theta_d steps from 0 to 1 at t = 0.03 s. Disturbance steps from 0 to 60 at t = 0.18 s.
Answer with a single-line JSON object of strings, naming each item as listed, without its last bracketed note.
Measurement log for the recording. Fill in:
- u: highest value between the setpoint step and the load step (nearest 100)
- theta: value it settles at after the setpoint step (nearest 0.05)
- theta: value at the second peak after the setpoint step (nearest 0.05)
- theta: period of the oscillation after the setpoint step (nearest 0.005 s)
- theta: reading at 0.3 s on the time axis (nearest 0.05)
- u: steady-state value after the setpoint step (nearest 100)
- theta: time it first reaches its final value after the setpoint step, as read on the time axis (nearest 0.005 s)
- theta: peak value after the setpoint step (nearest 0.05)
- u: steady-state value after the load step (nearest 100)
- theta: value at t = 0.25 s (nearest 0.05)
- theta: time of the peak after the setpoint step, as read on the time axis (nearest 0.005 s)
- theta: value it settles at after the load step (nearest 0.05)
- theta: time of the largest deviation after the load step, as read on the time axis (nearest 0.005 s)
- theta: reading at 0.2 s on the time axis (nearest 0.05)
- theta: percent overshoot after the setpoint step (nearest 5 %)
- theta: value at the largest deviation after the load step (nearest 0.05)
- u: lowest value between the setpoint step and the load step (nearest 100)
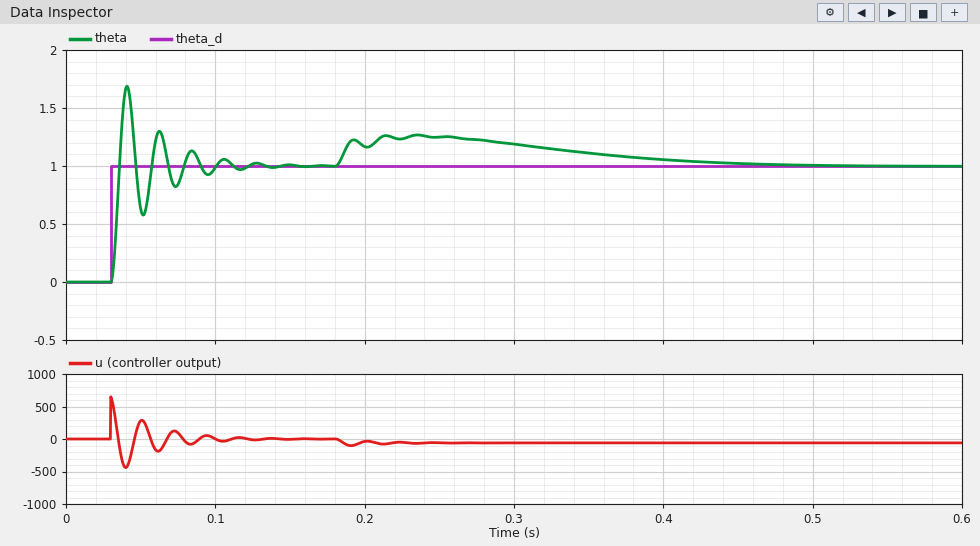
{"u: highest value between the setpoint step and the load step": "600", "theta: value it settles at after the setpoint step": "1.00", "theta: value at the second peak after the setpoint step": "1.30", "theta: period of the oscillation after the setpoint step": "0.020 s", "theta: reading at 0.3 s on the time axis": "1.20", "u: steady-state value after the setpoint step": "0", "theta: time it first reaches its final value after the setpoint step, as read on the time axis": "0.035 s", "theta: peak value after the setpoint step": "1.70", "u: steady-state value after the load step": "-100", "theta: value at t = 0.25 s": "1.25", "theta: time of the peak after the setpoint step, as read on the time axis": "0.040 s", "theta: value it settles at after the load step": "1.00", "theta: time of the largest deviation after the load step, as read on the time axis": "0.235 s", "theta: reading at 0.2 s on the time axis": "1.15", "theta: percent overshoot after the setpoint step": "70 %", "theta: value at the largest deviation after the load step": "1.25", "u: lowest value between the setpoint step and the load step": "-400"}
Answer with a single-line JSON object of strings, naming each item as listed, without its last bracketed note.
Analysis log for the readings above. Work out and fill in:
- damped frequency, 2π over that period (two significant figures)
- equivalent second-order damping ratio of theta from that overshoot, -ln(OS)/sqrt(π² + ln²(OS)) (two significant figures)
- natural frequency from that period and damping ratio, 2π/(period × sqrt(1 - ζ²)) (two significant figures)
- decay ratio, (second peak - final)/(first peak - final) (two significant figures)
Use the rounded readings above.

{"damped frequency, 2π over that period": "310 rad/s", "equivalent second-order damping ratio of theta from that overshoot, -ln(OS)/sqrt(π² + ln²(OS))": "0.11", "natural frequency from that period and damping ratio, 2π/(period × sqrt(1 - ζ²))": "320 rad/s", "decay ratio, (second peak - final)/(first peak - final)": "0.43"}
